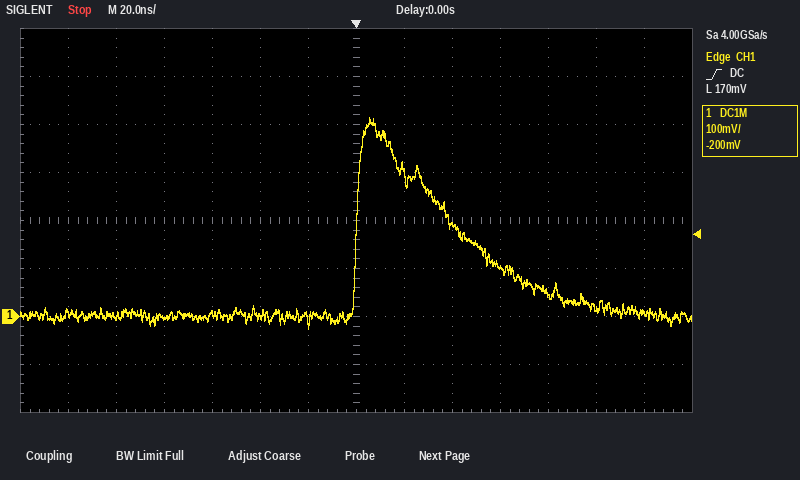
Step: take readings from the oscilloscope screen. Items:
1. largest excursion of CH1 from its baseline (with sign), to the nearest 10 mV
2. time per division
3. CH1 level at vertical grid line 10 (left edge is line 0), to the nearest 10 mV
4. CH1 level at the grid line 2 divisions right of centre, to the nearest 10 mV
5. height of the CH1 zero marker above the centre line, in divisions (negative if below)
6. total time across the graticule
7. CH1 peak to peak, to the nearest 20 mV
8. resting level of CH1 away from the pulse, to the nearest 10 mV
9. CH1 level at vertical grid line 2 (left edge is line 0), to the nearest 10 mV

+410 mV
20 ns
100 mV
190 mV
-2.0 div
280 ns
440 mV
0 mV
0 mV
